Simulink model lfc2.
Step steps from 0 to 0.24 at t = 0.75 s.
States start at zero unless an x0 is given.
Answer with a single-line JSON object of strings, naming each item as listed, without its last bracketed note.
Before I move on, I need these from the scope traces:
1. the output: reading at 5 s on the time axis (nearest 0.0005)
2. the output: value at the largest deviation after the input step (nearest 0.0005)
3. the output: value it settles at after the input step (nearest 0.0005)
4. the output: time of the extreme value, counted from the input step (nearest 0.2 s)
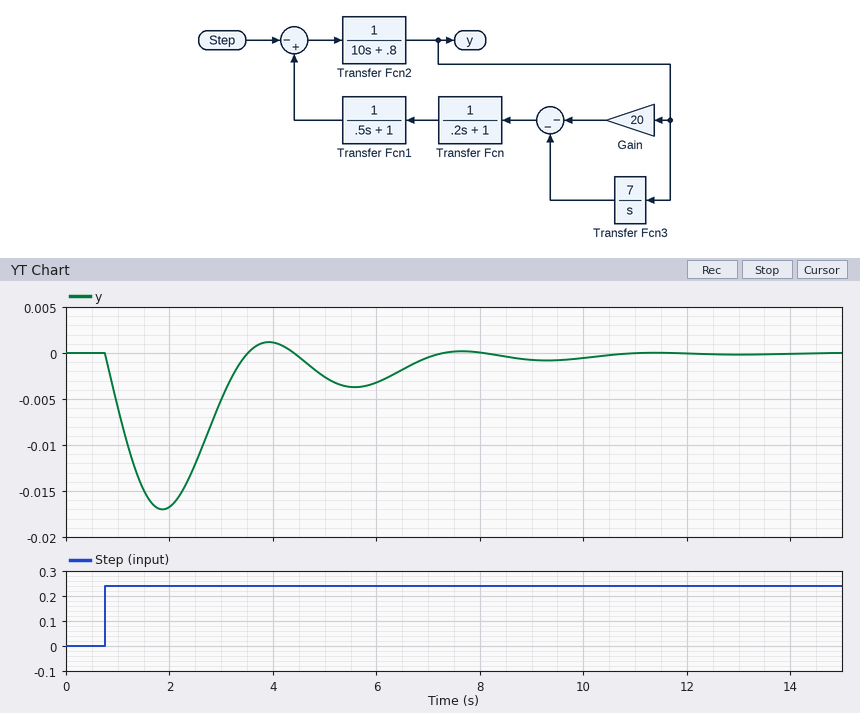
{"the output: reading at 5 s on the time axis": "-0.0025", "the output: value at the largest deviation after the input step": "-0.0170", "the output: value it settles at after the input step": "0.0000", "the output: time of the extreme value, counted from the input step": "1.2 s"}
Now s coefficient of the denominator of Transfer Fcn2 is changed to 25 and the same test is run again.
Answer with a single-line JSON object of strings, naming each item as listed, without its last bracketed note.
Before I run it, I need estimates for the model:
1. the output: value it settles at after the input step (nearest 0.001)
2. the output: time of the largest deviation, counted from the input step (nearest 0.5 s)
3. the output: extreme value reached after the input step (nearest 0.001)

{"the output: value it settles at after the input step": "0.000", "the output: time of the largest deviation, counted from the input step": "2.0 s", "the output: extreme value reached after the input step": "-0.011"}
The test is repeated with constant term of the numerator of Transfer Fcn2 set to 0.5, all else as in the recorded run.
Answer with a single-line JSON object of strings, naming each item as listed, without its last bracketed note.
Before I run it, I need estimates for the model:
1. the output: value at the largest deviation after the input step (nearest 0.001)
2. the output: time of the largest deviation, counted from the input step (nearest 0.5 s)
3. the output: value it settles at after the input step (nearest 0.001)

{"the output: value at the largest deviation after the input step": "-0.012", "the output: time of the largest deviation, counted from the input step": "1.5 s", "the output: value it settles at after the input step": "0.000"}
